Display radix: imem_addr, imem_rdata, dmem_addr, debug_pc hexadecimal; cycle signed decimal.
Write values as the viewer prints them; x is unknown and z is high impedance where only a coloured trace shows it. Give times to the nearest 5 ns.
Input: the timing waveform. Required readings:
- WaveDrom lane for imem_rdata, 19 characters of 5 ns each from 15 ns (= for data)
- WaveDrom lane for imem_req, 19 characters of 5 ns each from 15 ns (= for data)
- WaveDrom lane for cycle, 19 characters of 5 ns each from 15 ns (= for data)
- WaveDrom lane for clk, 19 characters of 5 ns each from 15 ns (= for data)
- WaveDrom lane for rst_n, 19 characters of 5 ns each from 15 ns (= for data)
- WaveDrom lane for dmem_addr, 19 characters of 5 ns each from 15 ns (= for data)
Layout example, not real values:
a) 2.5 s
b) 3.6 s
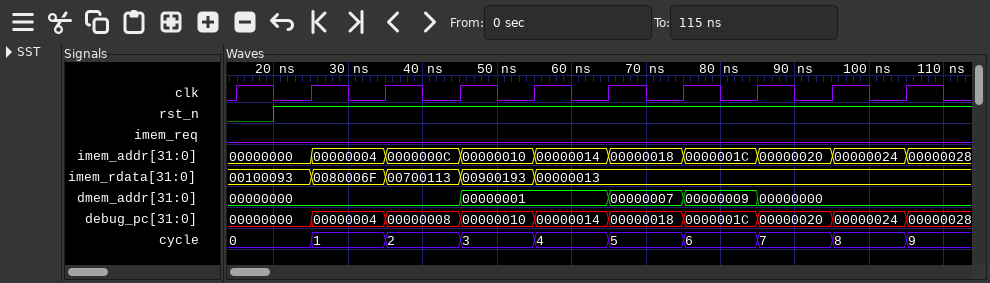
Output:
a) {name: 'imem_rdata', wave: '=.=.=.=.=..........', data: '00100093 0080006F 00700113 00900193 00000013'}
b) {name: 'imem_req', wave: '0..................'}
c) {name: 'cycle', wave: '=.=.=.=.=.=.=.=.=.=', data: '0 1 2 3 4 5 6 7 8 9'}
d) {name: 'clk', wave: '1010101010101010101'}
e) {name: 'rst_n', wave: '01.................'}
f) {name: 'dmem_addr', wave: '=.....=...=.=.=....', data: '00000000 00000001 00000007 00000009 00000000'}
